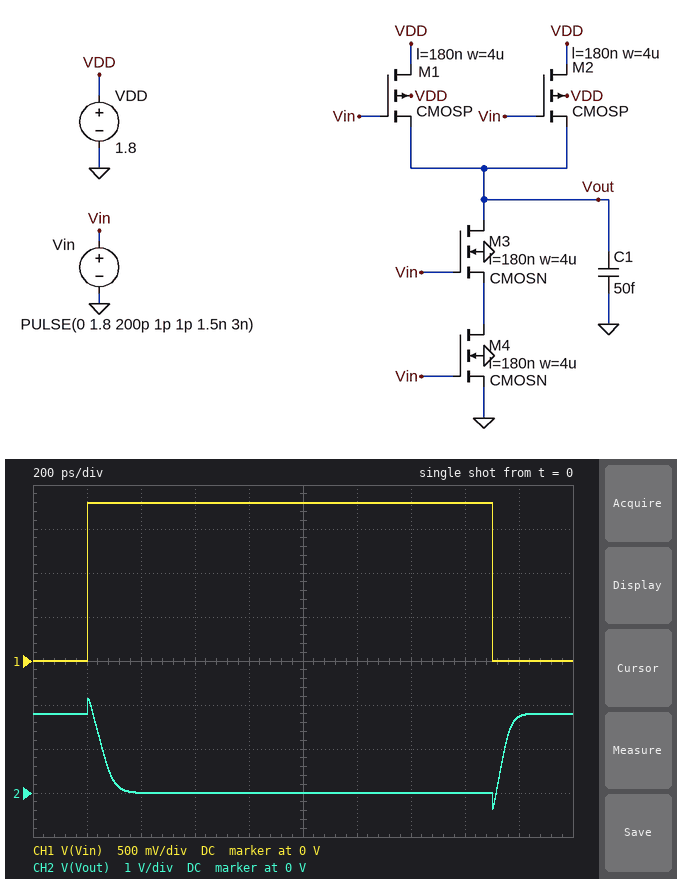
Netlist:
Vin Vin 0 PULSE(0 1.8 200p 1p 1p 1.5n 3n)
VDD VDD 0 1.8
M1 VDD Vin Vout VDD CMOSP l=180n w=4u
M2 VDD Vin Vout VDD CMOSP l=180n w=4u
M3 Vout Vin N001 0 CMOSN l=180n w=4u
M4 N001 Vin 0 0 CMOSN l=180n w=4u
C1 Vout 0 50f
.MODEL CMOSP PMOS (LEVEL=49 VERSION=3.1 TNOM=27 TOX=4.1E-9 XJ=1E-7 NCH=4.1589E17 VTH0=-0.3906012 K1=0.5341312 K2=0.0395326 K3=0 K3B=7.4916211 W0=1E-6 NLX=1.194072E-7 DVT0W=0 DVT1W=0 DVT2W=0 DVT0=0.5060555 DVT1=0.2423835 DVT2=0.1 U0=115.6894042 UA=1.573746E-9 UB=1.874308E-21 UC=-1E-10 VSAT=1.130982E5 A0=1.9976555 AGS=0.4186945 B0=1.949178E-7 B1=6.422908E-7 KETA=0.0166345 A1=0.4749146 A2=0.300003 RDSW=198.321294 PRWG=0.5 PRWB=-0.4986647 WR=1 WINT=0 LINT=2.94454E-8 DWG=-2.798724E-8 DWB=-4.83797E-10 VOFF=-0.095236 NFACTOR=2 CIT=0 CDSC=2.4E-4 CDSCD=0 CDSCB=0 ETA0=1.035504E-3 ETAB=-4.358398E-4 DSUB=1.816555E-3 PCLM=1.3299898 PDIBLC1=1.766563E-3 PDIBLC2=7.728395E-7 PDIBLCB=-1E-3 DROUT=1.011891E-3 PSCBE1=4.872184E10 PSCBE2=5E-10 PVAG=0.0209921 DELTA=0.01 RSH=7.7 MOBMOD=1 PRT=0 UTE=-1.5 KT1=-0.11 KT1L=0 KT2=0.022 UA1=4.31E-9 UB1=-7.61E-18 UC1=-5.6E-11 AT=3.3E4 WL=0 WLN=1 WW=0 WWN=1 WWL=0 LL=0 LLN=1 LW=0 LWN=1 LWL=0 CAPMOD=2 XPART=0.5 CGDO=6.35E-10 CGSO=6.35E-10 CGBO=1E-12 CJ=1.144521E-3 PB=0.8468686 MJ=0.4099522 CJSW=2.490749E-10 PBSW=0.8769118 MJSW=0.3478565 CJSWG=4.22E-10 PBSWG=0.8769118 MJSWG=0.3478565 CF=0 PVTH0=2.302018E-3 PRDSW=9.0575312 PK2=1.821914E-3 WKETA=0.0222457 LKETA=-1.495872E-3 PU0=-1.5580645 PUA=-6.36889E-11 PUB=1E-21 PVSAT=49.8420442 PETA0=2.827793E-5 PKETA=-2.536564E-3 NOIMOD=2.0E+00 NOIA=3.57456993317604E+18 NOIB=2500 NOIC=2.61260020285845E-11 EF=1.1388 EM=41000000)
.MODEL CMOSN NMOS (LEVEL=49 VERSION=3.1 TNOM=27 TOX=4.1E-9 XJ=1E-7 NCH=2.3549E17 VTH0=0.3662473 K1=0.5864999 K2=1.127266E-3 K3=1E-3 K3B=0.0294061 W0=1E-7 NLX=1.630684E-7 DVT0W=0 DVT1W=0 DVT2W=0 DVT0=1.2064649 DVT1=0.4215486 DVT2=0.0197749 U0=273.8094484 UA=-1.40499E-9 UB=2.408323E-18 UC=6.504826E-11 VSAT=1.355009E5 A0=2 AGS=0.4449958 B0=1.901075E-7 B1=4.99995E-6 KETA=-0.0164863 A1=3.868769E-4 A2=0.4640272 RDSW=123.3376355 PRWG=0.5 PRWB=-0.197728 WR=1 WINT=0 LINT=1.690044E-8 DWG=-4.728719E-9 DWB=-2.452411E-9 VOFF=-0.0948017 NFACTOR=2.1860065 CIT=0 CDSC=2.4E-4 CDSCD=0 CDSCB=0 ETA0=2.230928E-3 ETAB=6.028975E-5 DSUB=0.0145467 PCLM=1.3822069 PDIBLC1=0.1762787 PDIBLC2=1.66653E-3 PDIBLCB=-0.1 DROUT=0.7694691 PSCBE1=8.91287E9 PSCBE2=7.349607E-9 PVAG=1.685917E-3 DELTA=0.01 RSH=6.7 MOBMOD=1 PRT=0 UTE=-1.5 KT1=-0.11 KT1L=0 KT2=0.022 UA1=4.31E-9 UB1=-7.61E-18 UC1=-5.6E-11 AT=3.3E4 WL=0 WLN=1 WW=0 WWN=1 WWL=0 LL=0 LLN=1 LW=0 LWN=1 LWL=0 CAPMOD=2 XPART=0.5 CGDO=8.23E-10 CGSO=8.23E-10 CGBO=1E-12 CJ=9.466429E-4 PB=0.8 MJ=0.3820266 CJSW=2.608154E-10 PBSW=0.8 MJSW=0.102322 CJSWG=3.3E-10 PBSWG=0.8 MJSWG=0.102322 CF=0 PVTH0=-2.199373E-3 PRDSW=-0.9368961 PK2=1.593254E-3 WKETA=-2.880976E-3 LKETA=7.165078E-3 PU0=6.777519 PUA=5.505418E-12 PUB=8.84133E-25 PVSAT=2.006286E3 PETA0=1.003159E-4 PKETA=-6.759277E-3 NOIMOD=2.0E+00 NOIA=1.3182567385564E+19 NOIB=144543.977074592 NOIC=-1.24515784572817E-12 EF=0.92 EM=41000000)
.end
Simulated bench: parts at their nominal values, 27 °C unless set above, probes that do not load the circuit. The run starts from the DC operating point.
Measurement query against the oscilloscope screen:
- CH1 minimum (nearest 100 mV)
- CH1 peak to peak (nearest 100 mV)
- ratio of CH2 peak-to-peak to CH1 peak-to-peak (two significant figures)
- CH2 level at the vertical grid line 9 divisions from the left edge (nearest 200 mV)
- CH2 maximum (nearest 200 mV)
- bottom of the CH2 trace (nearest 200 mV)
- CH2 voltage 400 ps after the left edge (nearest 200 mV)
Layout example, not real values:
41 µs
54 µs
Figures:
0 V
1.8 V
1.4
1.8 V
2.2 V
-400 mV
0 V
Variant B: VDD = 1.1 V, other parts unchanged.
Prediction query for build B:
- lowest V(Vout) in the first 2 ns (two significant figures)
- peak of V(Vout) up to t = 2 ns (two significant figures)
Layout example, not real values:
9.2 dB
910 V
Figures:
-370 mV
1.4 V
